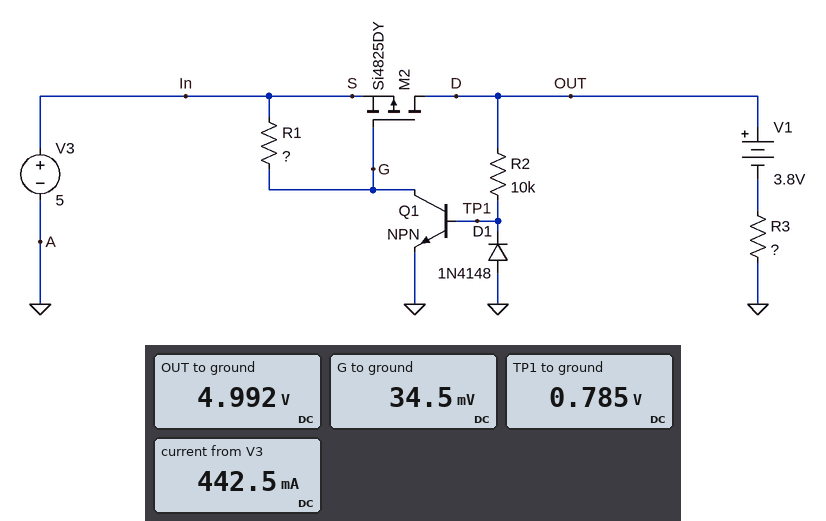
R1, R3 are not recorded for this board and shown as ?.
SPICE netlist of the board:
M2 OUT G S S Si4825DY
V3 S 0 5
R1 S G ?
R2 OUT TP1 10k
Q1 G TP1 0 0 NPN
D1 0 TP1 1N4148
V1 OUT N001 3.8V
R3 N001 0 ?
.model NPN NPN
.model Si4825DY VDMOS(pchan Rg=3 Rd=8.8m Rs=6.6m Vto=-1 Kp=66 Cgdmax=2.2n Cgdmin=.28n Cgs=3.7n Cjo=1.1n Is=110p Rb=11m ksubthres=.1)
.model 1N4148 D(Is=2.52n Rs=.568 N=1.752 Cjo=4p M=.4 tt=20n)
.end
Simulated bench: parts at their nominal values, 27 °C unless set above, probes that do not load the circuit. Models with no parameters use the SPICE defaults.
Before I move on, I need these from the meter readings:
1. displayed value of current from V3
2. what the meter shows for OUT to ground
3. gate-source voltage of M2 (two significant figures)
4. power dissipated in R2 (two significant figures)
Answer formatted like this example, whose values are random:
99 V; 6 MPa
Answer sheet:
442.5 mA; 4.992 V; -5.0 V; 1.8 mW
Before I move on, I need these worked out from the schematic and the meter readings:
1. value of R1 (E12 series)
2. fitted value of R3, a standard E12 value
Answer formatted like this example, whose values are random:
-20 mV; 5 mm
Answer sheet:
6.8 kΩ; 2.7 Ω
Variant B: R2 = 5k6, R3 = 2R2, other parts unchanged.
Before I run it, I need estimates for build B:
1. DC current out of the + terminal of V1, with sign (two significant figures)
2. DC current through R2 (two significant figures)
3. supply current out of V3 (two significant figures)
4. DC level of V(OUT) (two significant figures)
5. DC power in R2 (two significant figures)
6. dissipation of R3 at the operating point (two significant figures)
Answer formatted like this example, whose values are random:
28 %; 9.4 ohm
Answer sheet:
-540 mA; 750 µA; 540 mA; 5.0 V; 3.1 mW; 640 mW
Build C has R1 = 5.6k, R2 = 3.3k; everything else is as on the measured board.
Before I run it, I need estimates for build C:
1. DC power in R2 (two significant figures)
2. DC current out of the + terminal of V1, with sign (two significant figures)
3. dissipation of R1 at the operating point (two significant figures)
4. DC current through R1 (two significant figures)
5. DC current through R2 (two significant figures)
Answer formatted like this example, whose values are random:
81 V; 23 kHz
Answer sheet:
5.3 mW; -440 mA; 4.4 mW; 890 µA; 1.3 mA
